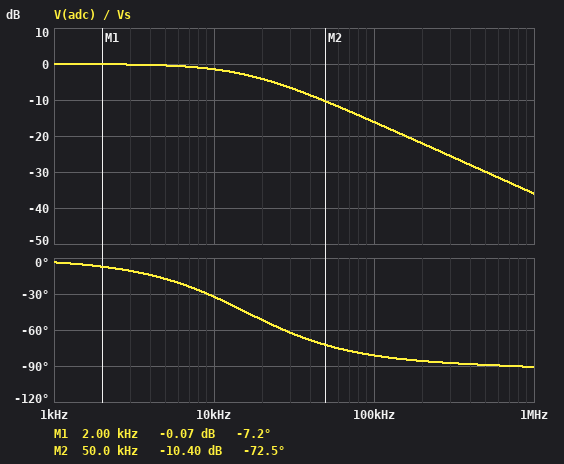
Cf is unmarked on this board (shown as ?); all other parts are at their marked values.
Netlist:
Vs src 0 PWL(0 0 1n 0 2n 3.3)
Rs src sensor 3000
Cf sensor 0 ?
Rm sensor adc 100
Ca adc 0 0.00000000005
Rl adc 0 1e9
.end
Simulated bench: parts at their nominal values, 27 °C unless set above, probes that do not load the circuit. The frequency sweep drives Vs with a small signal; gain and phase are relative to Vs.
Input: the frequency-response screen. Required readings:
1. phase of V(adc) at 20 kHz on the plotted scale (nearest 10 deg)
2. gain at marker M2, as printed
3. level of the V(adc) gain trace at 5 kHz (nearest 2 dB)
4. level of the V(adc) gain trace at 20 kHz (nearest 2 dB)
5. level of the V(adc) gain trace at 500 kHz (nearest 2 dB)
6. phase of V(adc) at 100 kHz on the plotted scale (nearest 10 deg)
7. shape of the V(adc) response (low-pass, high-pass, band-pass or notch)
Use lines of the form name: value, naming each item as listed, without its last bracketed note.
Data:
phase of V(adc) at 20 kHz on the plotted scale: -50 deg
gain at marker M2, as printed: -10.40 dB
level of the V(adc) gain trace at 5 kHz: 0 dB
level of the V(adc) gain trace at 20 kHz: -4 dB
level of the V(adc) gain trace at 500 kHz: -30 dB
phase of V(adc) at 100 kHz on the plotted scale: -80 deg
shape of the V(adc) response: low-pass
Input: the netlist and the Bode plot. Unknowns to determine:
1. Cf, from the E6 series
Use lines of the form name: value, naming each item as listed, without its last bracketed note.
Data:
Cf, from the E6 series: 3.3 nF
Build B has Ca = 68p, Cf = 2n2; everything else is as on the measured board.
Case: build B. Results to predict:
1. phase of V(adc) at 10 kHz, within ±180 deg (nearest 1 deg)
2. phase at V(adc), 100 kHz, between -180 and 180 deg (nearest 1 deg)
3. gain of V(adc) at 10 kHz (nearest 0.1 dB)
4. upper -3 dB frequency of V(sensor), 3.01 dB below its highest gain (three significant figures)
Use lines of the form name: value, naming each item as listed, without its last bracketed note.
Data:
phase of V(adc) at 10 kHz, within ±180 deg: -23 deg
phase at V(adc), 100 kHz, between -180 and 180 deg: -77 deg
gain of V(adc) at 10 kHz: -0.7 dB
upper -3 dB frequency of V(sensor), 3.01 dB below its highest gain: 23.4 kHz
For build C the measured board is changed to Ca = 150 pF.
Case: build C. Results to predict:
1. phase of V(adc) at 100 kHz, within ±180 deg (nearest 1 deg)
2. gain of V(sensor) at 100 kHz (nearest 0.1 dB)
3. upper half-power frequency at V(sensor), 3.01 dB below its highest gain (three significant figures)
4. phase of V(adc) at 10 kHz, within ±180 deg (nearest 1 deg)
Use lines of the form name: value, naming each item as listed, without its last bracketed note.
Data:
phase of V(adc) at 100 kHz, within ±180 deg: -82 deg
gain of V(sensor) at 100 kHz: -16.4 dB
upper half-power frequency at V(sensor), 3.01 dB below its highest gain: 15.4 kHz
phase of V(adc) at 10 kHz, within ±180 deg: -33 deg
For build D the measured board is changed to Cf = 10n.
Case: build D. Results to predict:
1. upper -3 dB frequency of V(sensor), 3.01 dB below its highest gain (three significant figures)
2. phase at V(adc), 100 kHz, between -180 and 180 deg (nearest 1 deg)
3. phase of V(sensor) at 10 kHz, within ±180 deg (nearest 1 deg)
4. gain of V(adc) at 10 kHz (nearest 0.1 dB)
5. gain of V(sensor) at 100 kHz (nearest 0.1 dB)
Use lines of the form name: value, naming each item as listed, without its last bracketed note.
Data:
upper -3 dB frequency of V(sensor), 3.01 dB below its highest gain: 5.28 kHz
phase at V(adc), 100 kHz, between -180 and 180 deg: -87 deg
phase of V(sensor) at 10 kHz, within ±180 deg: -62 deg
gain of V(adc) at 10 kHz: -6.6 dB
gain of V(sensor) at 100 kHz: -25.6 dB
